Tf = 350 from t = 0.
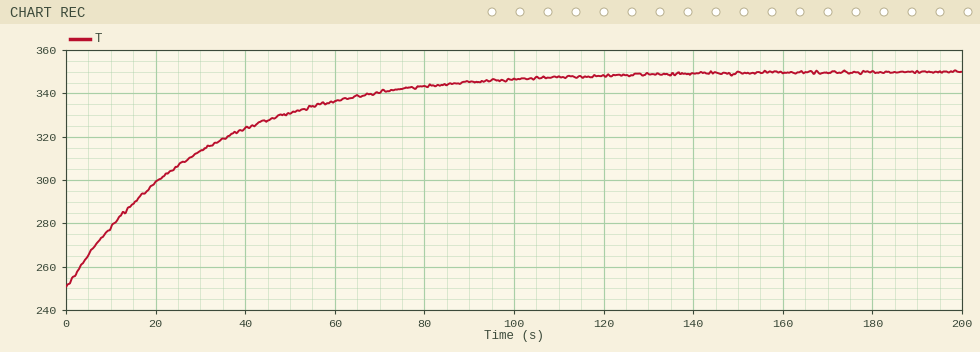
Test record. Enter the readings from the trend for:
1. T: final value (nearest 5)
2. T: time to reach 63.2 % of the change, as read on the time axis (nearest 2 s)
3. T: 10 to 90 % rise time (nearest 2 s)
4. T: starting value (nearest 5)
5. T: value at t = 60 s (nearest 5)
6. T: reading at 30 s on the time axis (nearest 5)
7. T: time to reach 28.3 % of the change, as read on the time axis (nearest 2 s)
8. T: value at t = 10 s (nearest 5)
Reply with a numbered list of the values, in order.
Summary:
1. 350
2. 30 s
3. 66 s
4. 250
5. 335
6. 315
7. 10 s
8. 280
